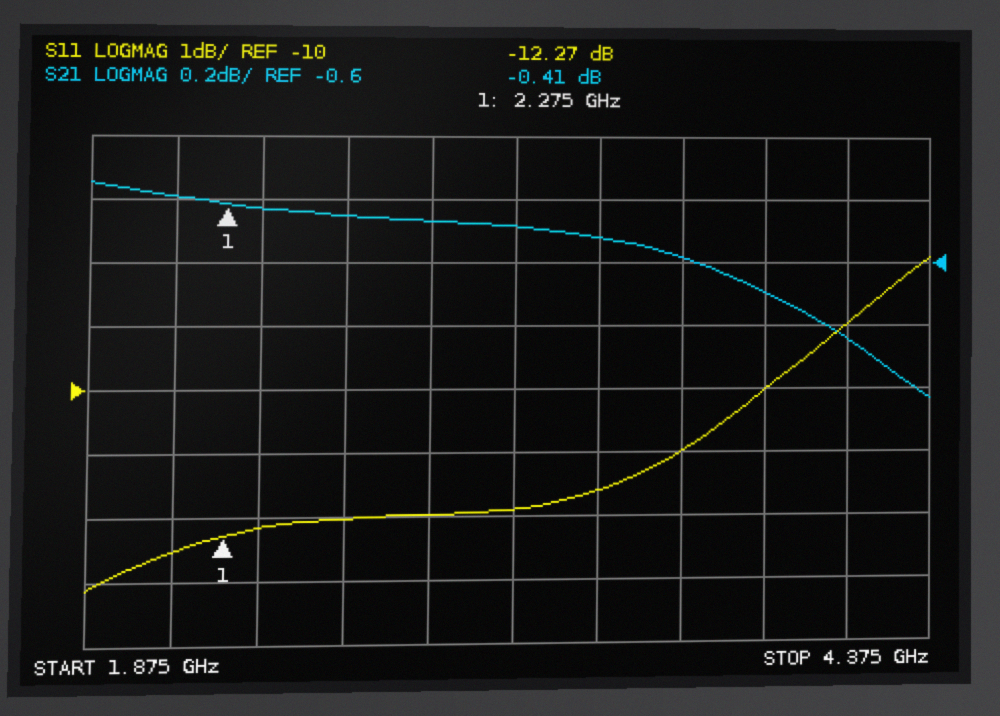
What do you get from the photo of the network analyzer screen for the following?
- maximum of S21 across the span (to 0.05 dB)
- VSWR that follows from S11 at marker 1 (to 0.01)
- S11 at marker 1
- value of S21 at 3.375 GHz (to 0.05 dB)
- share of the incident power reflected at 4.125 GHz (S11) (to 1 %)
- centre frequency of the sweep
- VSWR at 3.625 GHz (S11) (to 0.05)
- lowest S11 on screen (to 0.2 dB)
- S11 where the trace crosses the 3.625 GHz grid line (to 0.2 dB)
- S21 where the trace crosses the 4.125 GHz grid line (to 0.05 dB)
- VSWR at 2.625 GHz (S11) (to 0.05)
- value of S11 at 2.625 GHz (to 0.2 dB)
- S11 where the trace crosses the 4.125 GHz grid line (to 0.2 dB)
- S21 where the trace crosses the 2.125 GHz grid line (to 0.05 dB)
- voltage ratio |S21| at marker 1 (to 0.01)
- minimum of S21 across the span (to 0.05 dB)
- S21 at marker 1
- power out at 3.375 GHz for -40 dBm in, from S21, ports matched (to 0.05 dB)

-0.35 dB
1.64
-12.27 dB
-0.50 dB
13 %
3.125 GHz
1.80
-13.2 dB
-11.0 dB
-0.85 dB
1.65
-12.0 dB
-9.0 dB
-0.40 dB
0.95
-1.05 dB
-0.41 dB
-40.50 dBm
